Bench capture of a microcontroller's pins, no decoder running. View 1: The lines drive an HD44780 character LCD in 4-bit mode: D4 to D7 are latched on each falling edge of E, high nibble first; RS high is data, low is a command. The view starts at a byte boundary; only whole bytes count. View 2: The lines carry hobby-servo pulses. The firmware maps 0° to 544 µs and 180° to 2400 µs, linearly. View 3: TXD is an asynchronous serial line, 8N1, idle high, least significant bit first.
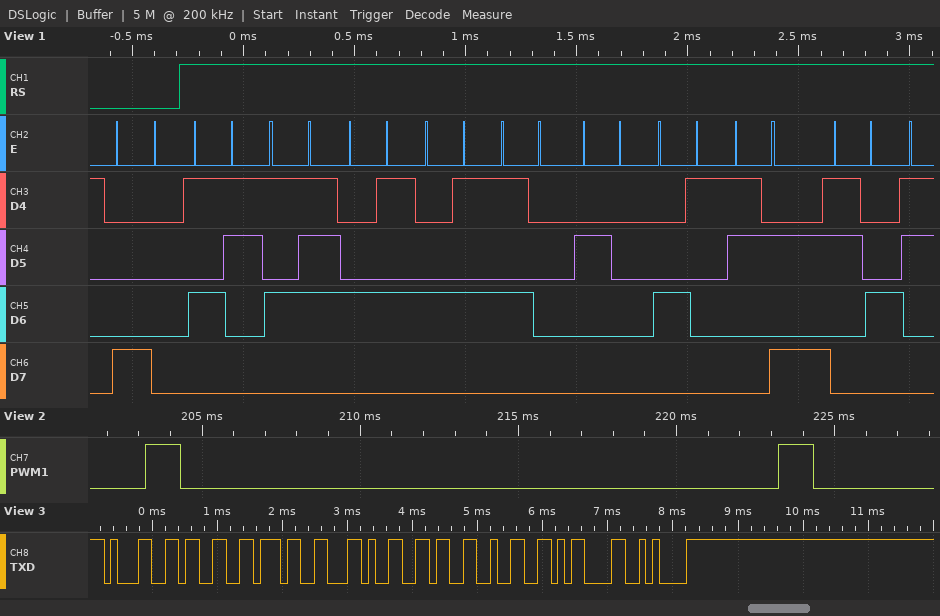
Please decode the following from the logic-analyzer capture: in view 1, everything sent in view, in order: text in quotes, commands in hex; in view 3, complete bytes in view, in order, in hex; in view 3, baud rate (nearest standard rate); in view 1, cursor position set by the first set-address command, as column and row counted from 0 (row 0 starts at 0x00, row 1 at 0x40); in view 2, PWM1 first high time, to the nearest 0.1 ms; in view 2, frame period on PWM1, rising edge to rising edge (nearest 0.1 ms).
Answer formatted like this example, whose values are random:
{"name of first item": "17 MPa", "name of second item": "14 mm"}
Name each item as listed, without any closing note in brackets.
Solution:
{"in view 1, everything sent in view, in order: text in quotes, commands in hex": "0x80 \"SWEEP A:4\"", "in view 3, complete bytes in view, in order, in hex": "0x31 0x33 0x37 0x2C 0x36 0x32 0x0D 0x0A", "in view 3, baud rate": "9600 baud", "in view 1, cursor position set by the first set-address command, as column and row counted from 0": "column 0, row 0", "in view 2, PWM1 first high time, to the nearest 0.1 ms": "1.1 ms", "in view 2, frame period on PWM1, rising edge to rising edge": "20.0 ms"}
